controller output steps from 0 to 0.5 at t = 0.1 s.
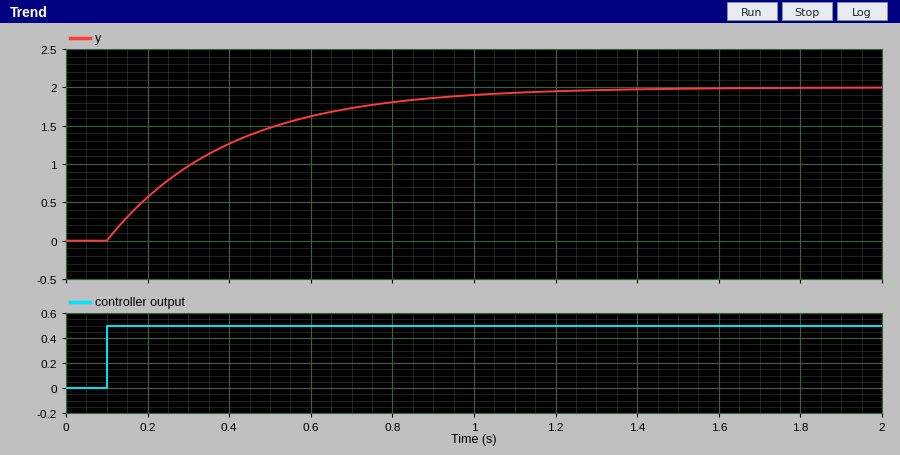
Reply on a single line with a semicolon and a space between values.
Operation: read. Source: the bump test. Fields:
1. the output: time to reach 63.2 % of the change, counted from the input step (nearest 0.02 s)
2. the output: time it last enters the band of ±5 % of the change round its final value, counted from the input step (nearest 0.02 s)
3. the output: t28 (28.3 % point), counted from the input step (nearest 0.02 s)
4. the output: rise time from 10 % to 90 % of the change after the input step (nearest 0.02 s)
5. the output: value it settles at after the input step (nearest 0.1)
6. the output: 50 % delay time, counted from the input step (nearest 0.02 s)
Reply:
0.30 s; 0.90 s; 0.10 s; 0.66 s; 2.0; 0.20 s
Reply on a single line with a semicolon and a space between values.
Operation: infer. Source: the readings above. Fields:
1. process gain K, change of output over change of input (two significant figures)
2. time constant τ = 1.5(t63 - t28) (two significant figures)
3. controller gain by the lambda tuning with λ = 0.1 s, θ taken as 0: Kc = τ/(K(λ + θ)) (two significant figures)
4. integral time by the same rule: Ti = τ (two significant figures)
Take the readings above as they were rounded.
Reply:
4.0; 0.30 s; 0.75; 0.30 s
